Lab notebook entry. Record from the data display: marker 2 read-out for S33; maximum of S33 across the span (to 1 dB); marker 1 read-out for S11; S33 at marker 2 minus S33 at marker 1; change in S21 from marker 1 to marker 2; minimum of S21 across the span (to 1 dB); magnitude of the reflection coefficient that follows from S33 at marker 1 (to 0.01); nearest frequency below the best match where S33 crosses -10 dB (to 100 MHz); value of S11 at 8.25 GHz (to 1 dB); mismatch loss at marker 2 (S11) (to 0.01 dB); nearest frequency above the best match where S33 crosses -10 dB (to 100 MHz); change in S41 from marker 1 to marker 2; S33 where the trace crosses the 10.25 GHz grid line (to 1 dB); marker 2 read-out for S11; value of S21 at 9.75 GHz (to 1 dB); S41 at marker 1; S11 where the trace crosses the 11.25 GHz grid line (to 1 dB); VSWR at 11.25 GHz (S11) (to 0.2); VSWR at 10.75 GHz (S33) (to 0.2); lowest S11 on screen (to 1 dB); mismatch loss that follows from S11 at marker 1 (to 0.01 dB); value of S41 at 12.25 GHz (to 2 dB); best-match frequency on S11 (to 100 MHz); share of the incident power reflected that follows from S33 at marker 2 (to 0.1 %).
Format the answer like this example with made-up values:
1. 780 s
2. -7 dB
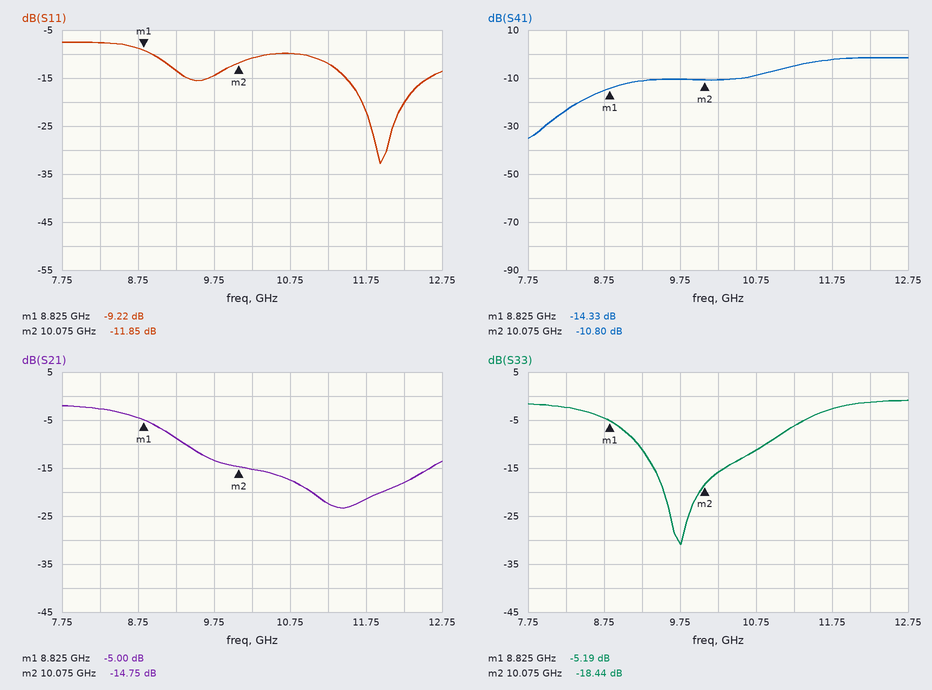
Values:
1. -18.44 dB
2. -1 dB
3. -9.22 dB
4. -13.25 dB
5. -9.75 dB
6. -23 dB
7. 0.55
8. 9.2 GHz
9. -8 dB
10. 0.29 dB
11. 10.9 GHz
12. 3.53 dB
13. -16 dB
14. -11.85 dB
15. -13 dB
16. -14.33 dB
17. -12 dB
18. 1.6
19. 1.8
20. -33 dB
21. 0.55 dB
22. -2 dB
23. 11.9 GHz
24. 1.4 %
